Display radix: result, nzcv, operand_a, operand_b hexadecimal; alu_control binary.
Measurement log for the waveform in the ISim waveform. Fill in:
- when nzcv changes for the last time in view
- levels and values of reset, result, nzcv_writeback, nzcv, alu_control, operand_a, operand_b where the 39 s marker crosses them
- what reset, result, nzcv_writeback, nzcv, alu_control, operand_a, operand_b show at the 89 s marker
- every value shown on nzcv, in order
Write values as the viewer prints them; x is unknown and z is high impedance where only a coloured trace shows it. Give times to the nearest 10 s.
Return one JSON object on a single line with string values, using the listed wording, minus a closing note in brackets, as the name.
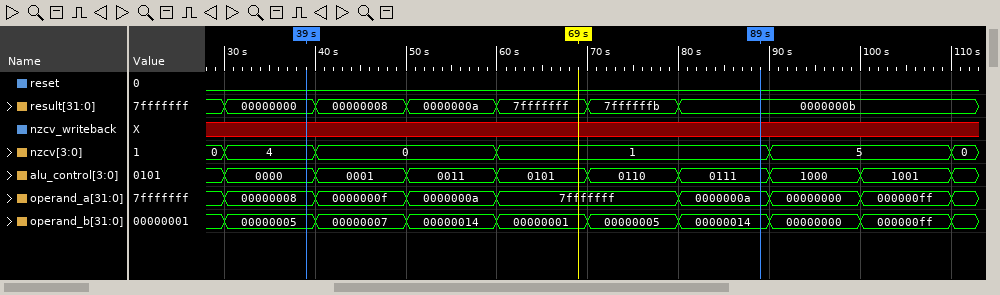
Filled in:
{"when nzcv changes for the last time in view": "110 s", "levels and values of reset, result, nzcv_writeback, nzcv, alu_control, operand_a, operand_b where the 39 s marker crosses them": "reset=0, result=00000000, nzcv_writeback=x, nzcv=4, alu_control=0000, operand_a=00000008, operand_b=00000005", "what reset, result, nzcv_writeback, nzcv, alu_control, operand_a, operand_b show at the 89 s marker": "reset=0, result=0000000b, nzcv_writeback=x, nzcv=1, alu_control=0111, operand_a=0000000a, operand_b=00000014", "every value shown on nzcv, in order": "0, 4, 0, 1, 5, 0"}
